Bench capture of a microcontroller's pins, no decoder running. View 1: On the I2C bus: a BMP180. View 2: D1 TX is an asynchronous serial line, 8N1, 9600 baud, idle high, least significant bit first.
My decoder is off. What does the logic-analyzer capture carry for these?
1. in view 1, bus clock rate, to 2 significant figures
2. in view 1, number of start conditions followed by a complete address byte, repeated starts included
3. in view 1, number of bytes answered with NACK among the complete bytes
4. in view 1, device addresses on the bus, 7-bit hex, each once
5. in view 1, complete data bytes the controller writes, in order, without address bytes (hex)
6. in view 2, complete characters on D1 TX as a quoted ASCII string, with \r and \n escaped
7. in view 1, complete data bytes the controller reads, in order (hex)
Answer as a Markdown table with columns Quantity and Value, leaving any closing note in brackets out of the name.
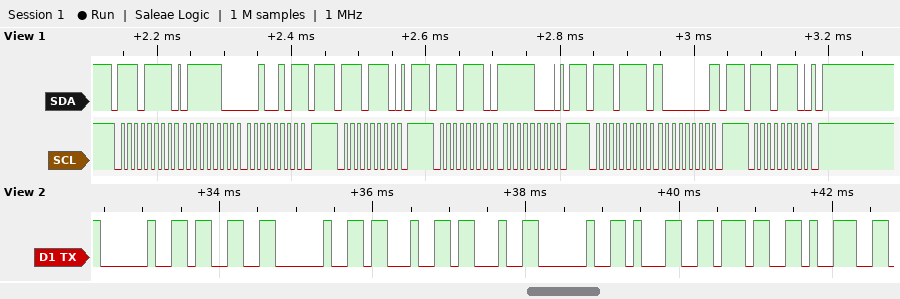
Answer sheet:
| Quantity | Value |
|---|---|
| in view 1, bus clock rate, to 2 significant figures | 100 kHz |
| in view 1, number of start conditions followed by a complete address byte, repeated starts included | 5 |
| in view 1, number of bytes answered with NACK among the complete bytes | 2 |
| in view 1, device addresses on the bus, 7-bit hex, each once | 0x77 |
| in view 1, complete data bytes the controller writes, in order, without address bytes | F8 |
| in view 2, complete characters on D1 TX as a quoted ASCII string, with \r and \n escaped | " 3 ## 179" |
| in view 1, complete data bytes the controller reads, in order | 7C 25 80 |
